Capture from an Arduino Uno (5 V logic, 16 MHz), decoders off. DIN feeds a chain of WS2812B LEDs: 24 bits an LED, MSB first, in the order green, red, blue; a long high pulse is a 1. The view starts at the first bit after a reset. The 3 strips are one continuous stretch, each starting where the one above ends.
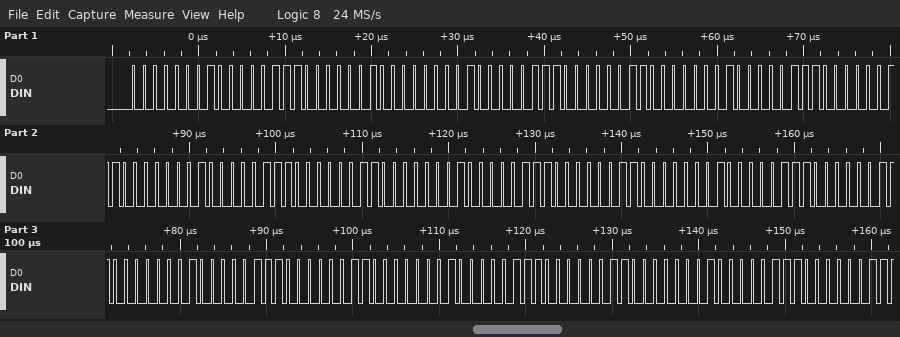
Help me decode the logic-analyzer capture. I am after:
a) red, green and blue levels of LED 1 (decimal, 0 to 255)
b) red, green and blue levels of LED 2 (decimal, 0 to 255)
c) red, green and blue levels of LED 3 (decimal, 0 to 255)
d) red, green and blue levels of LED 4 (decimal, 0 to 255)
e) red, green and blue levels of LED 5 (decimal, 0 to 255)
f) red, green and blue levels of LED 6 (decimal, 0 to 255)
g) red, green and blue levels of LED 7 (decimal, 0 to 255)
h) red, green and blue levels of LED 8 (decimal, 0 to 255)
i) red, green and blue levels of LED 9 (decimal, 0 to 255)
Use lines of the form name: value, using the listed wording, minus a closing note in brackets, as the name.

red, green and blue levels of LED 1: 7, 1, 2
red, green and blue levels of LED 2: 7, 1, 3
red, green and blue levels of LED 3: 7, 1, 3
red, green and blue levels of LED 4: 7, 1, 3
red, green and blue levels of LED 5: 7, 1, 3
red, green and blue levels of LED 6: 7, 1, 3
red, green and blue levels of LED 7: 7, 1, 3
red, green and blue levels of LED 8: 7, 1, 3
red, green and blue levels of LED 9: 7, 1, 3
